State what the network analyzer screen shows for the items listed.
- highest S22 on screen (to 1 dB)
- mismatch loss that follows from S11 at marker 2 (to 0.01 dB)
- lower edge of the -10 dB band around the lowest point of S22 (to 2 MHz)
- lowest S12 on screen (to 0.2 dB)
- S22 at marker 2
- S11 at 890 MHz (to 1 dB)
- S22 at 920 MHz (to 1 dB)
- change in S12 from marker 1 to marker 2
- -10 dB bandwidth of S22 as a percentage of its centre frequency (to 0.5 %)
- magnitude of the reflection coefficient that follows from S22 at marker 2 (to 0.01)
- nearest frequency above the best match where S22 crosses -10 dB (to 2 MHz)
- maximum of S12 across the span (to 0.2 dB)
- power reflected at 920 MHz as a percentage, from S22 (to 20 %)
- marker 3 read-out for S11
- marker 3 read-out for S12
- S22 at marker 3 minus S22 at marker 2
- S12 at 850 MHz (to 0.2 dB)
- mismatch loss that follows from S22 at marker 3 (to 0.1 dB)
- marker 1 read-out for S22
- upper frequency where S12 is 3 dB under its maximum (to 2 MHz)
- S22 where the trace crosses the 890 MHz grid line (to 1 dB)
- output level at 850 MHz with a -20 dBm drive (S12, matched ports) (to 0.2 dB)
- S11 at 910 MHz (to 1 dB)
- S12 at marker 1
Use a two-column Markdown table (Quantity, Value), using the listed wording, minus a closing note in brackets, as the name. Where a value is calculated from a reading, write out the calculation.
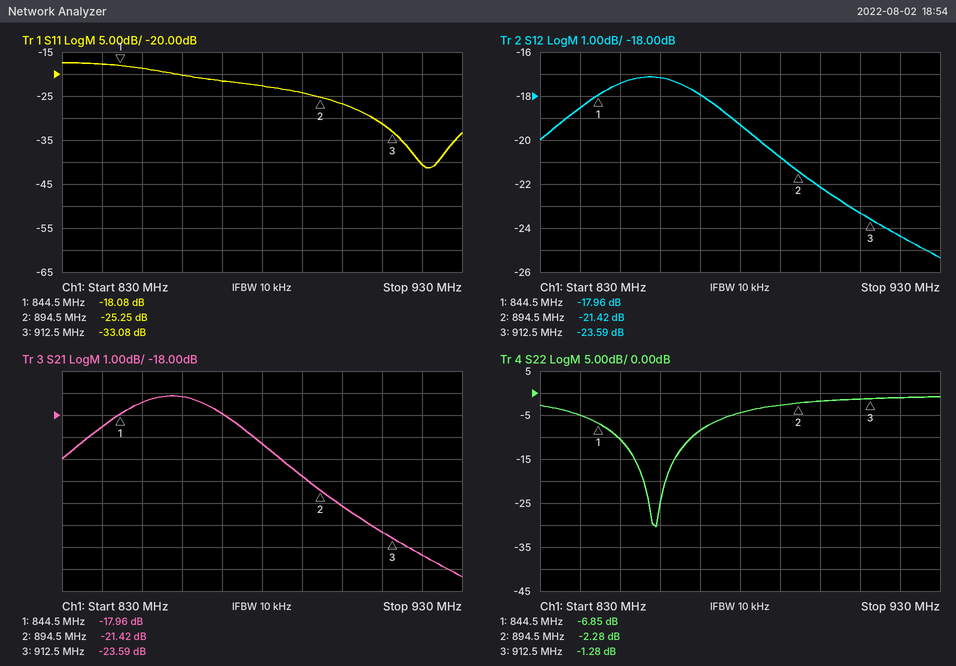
| Quantity | Value |
|---|---|
| highest S22 on screen | -1 dB |
| mismatch loss that follows from S11 at marker 2 | −10 log10(1 − 10^(-25.25/10)) ≈ 0.01 dB |
| lower edge of the -10 dB band around the lowest point of S22 | 850 MHz |
| lowest S12 on screen | -25.4 dB |
| S22 at marker 2 | -2.28 dB |
| S11 at 890 MHz | -24 dB |
| S22 at 920 MHz | -1 dB |
| change in S12 from marker 1 to marker 2 | -21.42 − (-17.96) = -3.46 dB |
| -10 dB bandwidth of S22 as a percentage of its centre frequency | 18 MHz / 859 MHz ≈ 2.10 %, so 2.0 % to the nearest 0.5 % |
| magnitude of the reflection coefficient that follows from S22 at marker 2 | 10^(-2.28/20) ≈ 0.77 |
| nearest frequency above the best match where S22 crosses -10 dB | 868 MHz |
| maximum of S12 across the span | -17.2 dB |
| power reflected at 920 MHz as a percentage, from S22 | 10^(-1/10) ≈ 79.4 %, so 80 % to the nearest 20 % |
| marker 3 read-out for S11 | -33.08 dB |
| marker 3 read-out for S12 | -23.59 dB |
| S22 at marker 3 minus S22 at marker 2 | -1.28 − (-2.28) = 1.00 dB |
| S12 at 850 MHz | -17.4 dB |
| mismatch loss that follows from S22 at marker 3 | −10 log10(1 − 10^(-1.28/10)) ≈ 5.9 dB |
| marker 1 read-out for S22 | -6.85 dB |
| upper frequency where S12 is 3 dB under its maximum | 886 MHz |
| S22 where the trace crosses the 890 MHz grid line | -3 dB |
| output level at 850 MHz with a -20 dBm drive (S12, matched ports) | -20 dBm + (-17.4 dB) = -37.4 dBm |
| S11 at 910 MHz | -31 dB |
| S12 at marker 1 | -17.96 dB |
